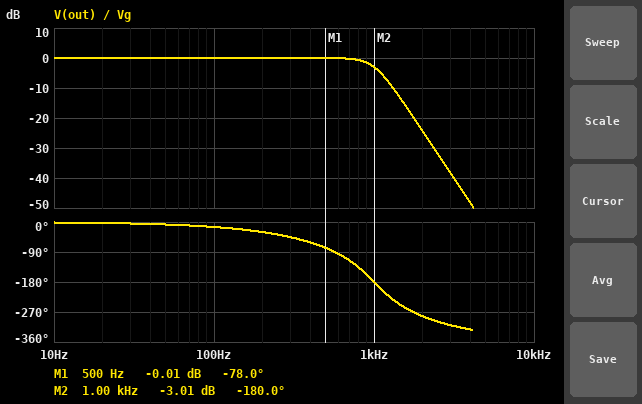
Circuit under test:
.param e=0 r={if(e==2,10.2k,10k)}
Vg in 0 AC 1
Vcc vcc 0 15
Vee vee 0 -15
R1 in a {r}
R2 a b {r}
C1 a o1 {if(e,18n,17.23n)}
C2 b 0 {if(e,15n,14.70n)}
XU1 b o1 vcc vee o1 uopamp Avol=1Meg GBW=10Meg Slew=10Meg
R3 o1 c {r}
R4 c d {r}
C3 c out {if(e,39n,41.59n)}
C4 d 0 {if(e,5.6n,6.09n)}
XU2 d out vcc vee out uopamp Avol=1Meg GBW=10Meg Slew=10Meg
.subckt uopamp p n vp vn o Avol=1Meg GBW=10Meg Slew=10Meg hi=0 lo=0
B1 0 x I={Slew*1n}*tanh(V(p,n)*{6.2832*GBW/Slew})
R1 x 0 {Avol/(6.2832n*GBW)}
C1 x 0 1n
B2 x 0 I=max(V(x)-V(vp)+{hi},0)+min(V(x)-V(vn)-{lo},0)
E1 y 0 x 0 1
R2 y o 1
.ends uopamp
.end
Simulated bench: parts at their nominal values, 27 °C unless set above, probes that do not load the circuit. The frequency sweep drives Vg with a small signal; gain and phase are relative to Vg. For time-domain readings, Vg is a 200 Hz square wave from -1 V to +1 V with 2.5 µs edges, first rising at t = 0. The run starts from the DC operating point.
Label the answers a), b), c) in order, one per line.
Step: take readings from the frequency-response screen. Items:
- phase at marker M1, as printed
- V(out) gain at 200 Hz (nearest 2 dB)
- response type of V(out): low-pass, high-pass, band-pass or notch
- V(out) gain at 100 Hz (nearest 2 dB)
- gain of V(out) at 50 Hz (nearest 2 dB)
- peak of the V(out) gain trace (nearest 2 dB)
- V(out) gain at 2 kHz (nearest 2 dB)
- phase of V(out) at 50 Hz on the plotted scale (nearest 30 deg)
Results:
a) -78.0 deg
b) 0 dB
c) low-pass
d) 0 dB
e) 0 dB
f) 0 dB
g) -24 dB
h) 0 deg
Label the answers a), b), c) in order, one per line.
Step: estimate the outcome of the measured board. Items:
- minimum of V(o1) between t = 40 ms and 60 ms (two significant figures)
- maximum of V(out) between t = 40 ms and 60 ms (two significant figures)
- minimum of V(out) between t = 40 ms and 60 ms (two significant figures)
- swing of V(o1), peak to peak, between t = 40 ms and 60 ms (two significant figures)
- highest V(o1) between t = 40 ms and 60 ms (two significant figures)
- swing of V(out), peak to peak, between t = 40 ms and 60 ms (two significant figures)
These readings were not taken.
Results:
a) -1.0 V
b) 1.2 V
c) -1.2 V
d) 2.0 V
e) 1.0 V
f) 2.4 V
